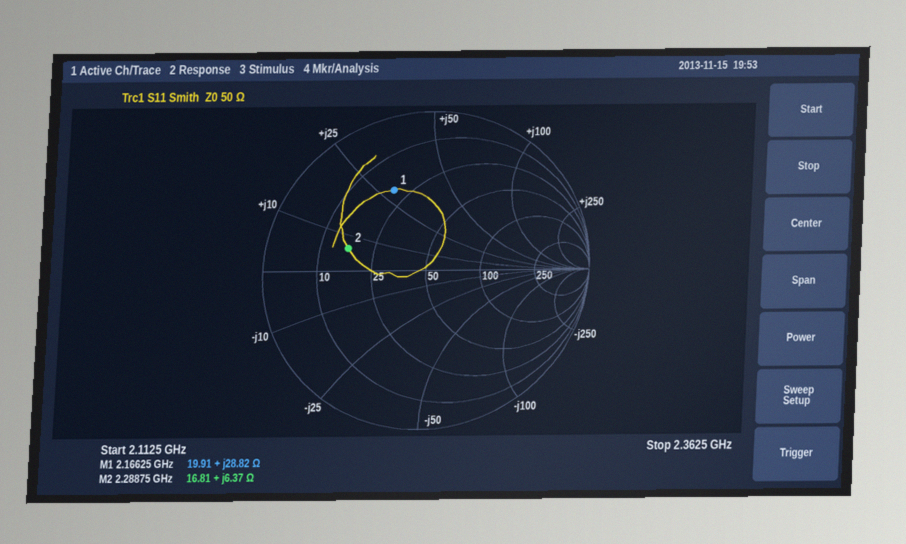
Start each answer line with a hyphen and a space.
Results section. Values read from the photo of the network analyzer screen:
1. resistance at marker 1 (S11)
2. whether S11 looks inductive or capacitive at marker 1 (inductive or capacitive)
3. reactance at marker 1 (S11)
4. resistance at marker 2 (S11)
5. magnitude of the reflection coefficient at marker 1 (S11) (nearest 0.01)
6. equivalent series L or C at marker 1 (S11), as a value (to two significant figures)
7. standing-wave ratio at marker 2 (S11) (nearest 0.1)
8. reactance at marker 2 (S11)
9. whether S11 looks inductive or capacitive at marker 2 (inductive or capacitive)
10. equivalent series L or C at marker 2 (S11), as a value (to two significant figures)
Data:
- 19.91 Ω
- inductive
- +28.82 Ω
- 16.81 Ω
- 0.55
- 2.1 nH
- 3.0
- +6.37 Ω
- inductive
- 440 pH
